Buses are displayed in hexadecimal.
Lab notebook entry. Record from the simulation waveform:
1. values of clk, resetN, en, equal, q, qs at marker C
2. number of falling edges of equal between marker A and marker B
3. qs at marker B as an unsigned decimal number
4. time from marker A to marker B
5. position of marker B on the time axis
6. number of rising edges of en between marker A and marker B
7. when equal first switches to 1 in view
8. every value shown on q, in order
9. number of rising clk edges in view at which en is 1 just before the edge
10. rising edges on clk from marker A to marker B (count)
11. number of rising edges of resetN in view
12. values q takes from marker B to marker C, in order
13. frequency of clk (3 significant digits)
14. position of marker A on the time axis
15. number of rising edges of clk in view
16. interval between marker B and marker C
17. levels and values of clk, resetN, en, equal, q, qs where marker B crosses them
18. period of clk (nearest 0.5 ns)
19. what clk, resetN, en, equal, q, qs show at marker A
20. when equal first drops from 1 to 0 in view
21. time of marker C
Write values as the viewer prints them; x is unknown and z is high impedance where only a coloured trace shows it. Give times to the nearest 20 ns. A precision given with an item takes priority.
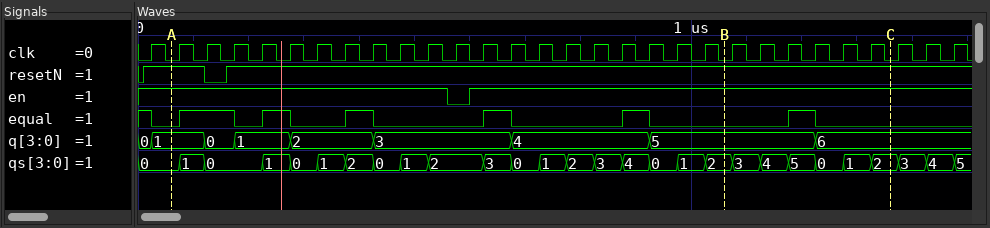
clk=0, resetN=1, en=1, equal=0, q=6, qs=2
5
2
1000 ns
1060 ns
1
80 ns
0, 1, 0, 1, 2, 3, 4, 5, 6
29
20
2
5, 6
20.0 MHz
60 ns
30
300 ns
clk=0, resetN=1, en=1, equal=0, q=5, qs=2
50 ns
clk=0, resetN=1, en=1, equal=0, q=1, qs=0
20 ns
1360 ns
